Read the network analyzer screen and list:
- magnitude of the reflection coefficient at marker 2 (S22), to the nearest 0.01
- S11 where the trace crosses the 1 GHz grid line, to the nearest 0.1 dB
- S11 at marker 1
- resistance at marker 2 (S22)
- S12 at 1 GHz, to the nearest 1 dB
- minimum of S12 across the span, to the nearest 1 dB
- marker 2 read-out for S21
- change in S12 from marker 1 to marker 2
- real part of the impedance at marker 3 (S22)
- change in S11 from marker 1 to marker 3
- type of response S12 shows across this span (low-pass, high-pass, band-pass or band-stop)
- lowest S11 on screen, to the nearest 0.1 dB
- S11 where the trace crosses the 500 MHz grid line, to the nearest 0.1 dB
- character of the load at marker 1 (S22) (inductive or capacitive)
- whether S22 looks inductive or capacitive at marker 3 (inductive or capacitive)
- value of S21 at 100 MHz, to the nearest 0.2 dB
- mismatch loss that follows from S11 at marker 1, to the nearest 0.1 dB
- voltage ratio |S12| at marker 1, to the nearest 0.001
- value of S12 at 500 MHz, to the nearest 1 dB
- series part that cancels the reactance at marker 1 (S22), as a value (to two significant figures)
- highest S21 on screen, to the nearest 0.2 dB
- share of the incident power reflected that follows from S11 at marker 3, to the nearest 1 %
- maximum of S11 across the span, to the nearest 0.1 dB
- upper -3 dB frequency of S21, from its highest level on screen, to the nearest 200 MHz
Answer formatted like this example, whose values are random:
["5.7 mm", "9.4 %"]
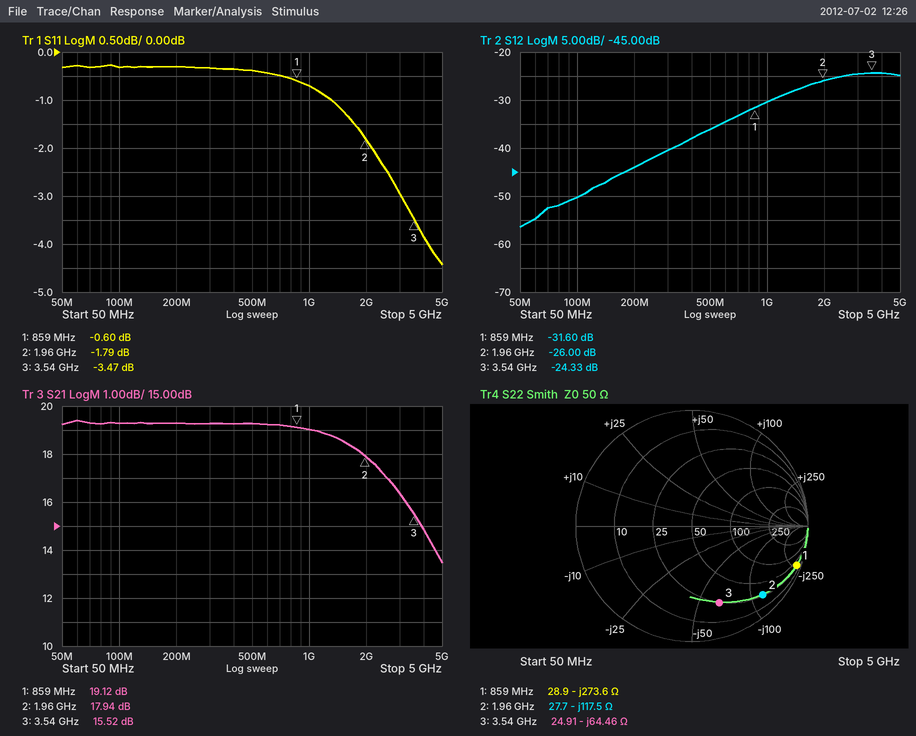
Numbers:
["0.85", "-0.7 dB", "-0.60 dB", "27.7 Ω", "-30 dB", "-56 dB", "17.94 dB", "5.60 dB", "24.91 Ω", "-2.87 dB", "high-pass", "-4.4 dB", "-0.4 dB", "capacitive", "capacitive", "19.2 dB", "8.9 dB", "0.026", "-36 dB", "51 nH", "19.4 dB", "45 %", "-0.3 dB", "3.0 GHz"]
